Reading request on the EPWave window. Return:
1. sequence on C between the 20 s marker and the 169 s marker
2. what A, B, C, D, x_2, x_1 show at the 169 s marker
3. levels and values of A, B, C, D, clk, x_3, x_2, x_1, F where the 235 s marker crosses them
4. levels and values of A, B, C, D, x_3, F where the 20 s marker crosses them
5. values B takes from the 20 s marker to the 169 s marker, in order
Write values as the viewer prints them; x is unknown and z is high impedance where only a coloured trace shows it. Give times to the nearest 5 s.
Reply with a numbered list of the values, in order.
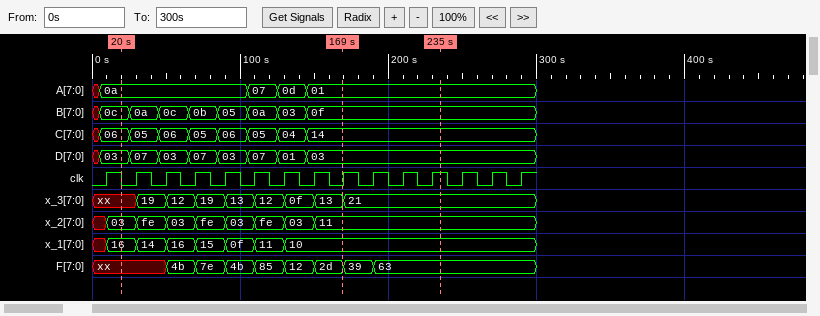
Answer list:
1. 06, 05, 06, 05, 06, 05, 04, 14
2. A=01, B=0f, C=14, D=03, x_2=11, x_1=10
3. A=01, B=0f, C=14, D=03, clk=1, x_3=21, x_2=11, x_1=10, F=63
4. A=0a, B=0c, C=06, D=03, x_3=xx, F=xx
5. 0c, 0a, 0c, 0b, 05, 0a, 03, 0f
